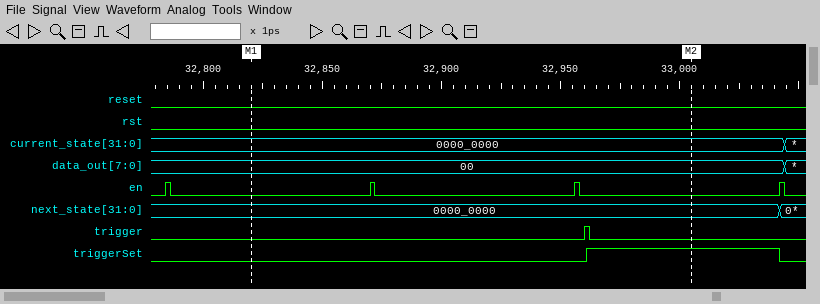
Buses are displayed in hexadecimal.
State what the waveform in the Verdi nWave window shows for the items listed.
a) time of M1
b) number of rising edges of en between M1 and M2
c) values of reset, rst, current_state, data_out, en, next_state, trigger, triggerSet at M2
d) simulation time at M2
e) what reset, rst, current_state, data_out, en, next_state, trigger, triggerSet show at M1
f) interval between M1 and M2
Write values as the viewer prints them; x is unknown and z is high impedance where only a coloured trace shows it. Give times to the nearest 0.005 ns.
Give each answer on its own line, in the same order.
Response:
32.82 ns
2
reset=0, rst=0, current_state=0000_0000, data_out=00, en=0, next_state=0000_0000, trigger=0, triggerSet=1
33.005 ns
reset=0, rst=0, current_state=0000_0000, data_out=00, en=0, next_state=0000_0000, trigger=0, triggerSet=0
0.185 ns
